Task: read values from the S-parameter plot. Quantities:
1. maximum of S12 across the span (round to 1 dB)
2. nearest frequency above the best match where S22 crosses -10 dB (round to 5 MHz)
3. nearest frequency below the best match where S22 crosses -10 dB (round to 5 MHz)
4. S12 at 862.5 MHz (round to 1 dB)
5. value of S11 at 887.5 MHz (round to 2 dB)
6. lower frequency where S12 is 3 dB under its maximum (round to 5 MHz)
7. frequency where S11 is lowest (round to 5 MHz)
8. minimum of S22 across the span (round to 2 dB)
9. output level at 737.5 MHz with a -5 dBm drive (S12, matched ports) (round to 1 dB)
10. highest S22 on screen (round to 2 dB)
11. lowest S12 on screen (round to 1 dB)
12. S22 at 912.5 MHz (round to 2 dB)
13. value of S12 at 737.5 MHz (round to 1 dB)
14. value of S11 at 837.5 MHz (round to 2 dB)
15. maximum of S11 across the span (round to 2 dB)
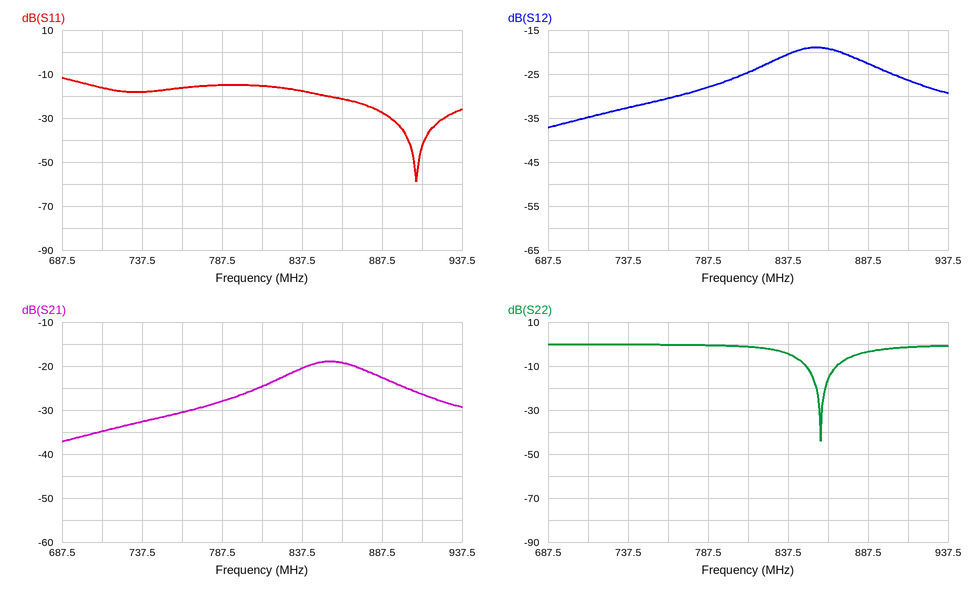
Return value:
-19 dB
870 MHz
850 MHz
-19 dB
-28 dB
830 MHz
910 MHz
-44 dB
-38 dBm
0 dB
-37 dB
-2 dB
-33 dB
-18 dB
-12 dB
